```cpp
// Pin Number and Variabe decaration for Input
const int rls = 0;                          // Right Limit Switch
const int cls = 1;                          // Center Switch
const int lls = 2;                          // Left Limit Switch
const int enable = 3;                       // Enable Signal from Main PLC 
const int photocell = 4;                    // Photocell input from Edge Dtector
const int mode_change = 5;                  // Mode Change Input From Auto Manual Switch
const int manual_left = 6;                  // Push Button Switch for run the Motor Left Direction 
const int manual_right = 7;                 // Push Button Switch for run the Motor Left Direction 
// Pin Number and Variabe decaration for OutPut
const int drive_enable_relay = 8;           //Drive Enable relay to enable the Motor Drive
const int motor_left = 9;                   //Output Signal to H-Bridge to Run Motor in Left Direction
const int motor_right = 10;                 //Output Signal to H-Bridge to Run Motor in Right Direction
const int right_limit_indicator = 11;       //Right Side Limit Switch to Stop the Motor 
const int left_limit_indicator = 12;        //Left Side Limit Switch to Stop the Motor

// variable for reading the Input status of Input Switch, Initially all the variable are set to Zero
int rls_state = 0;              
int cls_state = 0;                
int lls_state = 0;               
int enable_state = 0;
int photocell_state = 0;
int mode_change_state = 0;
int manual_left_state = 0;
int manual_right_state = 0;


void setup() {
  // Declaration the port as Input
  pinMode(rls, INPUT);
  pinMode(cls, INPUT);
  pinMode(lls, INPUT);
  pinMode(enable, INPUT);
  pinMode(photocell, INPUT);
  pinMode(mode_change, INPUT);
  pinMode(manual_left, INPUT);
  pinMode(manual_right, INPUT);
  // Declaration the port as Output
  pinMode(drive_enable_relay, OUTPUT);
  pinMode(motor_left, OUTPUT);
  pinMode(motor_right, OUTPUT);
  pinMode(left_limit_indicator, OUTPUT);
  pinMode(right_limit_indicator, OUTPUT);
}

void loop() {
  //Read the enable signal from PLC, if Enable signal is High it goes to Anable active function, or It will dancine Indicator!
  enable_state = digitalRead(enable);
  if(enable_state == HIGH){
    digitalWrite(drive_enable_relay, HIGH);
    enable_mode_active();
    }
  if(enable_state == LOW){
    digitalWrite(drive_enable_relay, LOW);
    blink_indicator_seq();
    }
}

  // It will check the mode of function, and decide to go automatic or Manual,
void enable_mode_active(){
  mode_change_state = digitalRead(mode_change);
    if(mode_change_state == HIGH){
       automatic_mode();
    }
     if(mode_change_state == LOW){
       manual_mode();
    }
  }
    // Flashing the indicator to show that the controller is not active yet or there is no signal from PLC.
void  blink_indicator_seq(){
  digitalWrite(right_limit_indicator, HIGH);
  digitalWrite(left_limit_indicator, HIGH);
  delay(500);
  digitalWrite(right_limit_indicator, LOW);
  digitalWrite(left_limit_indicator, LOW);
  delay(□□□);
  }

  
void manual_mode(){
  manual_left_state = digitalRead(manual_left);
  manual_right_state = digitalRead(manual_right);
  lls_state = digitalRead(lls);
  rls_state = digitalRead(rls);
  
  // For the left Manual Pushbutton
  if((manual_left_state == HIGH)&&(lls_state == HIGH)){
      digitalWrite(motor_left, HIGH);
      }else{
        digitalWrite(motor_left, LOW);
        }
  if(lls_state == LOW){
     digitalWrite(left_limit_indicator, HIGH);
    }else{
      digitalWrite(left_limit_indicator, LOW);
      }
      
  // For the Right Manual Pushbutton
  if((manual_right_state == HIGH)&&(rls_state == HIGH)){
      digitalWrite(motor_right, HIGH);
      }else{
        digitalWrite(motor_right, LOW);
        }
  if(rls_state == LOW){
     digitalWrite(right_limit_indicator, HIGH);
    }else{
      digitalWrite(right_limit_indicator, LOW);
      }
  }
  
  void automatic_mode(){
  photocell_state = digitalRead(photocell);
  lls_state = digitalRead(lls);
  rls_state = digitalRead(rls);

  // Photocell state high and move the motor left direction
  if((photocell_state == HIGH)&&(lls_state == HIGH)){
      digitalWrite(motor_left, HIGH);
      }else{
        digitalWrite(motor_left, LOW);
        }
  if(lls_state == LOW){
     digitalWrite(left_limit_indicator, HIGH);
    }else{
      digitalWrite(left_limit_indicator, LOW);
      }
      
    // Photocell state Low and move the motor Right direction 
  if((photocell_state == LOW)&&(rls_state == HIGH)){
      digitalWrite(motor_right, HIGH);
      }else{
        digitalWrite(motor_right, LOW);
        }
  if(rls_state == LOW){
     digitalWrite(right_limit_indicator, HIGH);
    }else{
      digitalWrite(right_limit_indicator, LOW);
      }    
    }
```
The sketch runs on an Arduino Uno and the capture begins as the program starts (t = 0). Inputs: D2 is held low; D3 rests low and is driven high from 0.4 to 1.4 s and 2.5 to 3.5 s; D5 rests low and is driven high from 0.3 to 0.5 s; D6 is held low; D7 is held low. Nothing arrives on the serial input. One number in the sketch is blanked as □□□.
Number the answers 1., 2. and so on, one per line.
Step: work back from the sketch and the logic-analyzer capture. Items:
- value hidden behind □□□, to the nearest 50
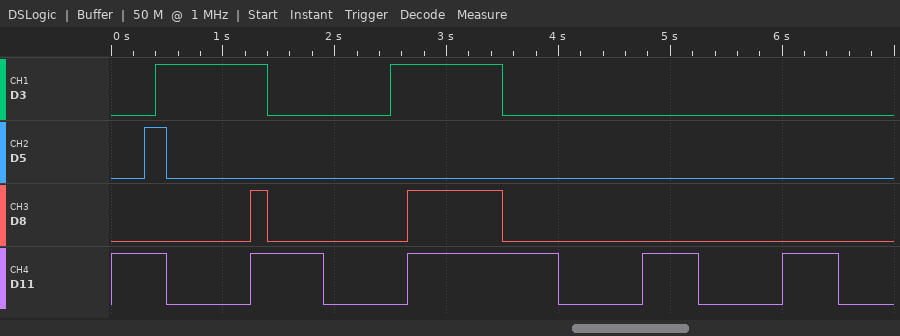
1. 750
